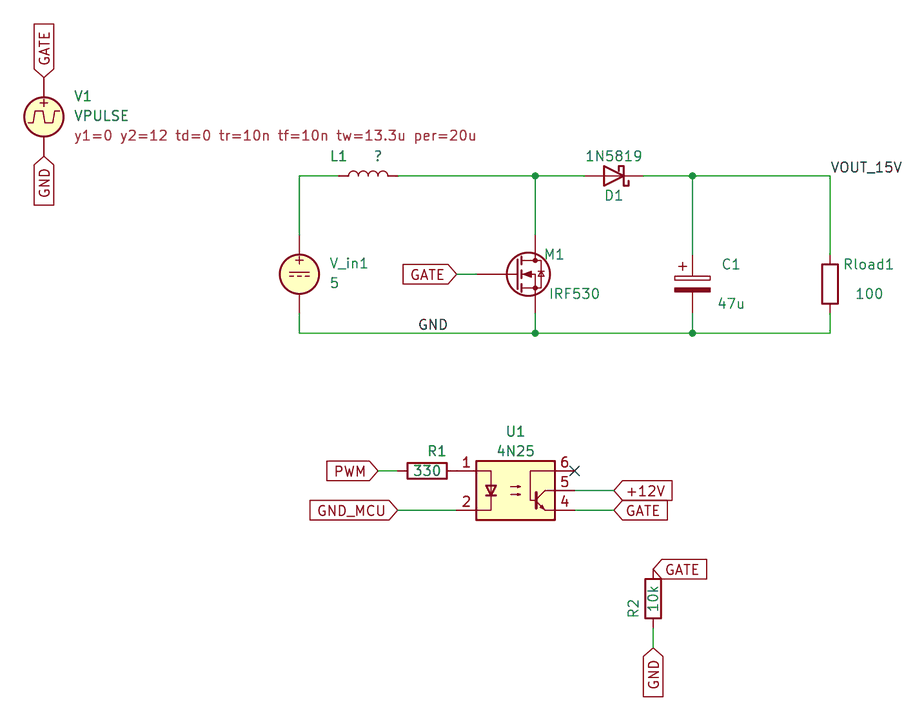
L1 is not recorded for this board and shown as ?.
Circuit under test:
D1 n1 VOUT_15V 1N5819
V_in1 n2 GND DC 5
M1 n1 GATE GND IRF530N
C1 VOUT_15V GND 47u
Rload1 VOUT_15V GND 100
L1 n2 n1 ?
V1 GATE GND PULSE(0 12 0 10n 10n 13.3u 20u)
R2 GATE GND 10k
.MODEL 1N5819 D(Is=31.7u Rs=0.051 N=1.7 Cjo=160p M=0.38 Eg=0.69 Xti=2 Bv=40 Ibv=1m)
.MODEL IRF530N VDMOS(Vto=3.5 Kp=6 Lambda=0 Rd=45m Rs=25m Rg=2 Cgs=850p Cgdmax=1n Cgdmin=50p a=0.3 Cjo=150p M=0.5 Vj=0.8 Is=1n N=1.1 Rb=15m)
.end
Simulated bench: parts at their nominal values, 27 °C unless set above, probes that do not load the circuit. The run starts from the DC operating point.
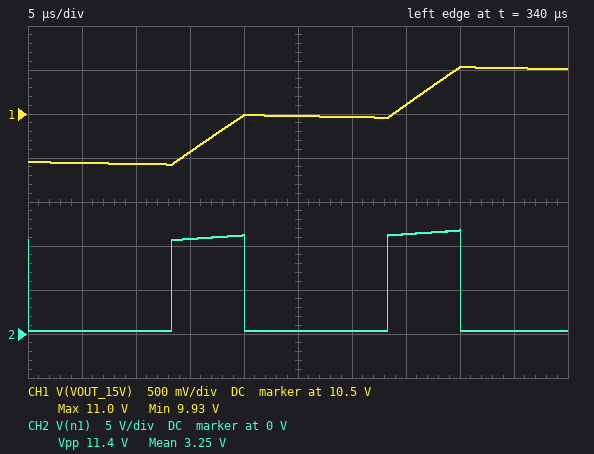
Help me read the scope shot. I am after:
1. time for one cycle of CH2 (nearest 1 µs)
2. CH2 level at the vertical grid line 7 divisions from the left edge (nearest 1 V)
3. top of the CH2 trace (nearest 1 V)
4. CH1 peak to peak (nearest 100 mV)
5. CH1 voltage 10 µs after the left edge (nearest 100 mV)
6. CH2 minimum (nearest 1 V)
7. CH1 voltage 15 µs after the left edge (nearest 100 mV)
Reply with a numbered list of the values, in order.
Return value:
1. 20 µs
2. 11 V
3. 12 V
4. 1.1 V
5. 9.9 V
6. 0 V
7. 10.1 V
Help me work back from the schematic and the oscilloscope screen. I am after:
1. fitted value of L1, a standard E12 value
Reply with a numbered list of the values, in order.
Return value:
1. 220 µH
